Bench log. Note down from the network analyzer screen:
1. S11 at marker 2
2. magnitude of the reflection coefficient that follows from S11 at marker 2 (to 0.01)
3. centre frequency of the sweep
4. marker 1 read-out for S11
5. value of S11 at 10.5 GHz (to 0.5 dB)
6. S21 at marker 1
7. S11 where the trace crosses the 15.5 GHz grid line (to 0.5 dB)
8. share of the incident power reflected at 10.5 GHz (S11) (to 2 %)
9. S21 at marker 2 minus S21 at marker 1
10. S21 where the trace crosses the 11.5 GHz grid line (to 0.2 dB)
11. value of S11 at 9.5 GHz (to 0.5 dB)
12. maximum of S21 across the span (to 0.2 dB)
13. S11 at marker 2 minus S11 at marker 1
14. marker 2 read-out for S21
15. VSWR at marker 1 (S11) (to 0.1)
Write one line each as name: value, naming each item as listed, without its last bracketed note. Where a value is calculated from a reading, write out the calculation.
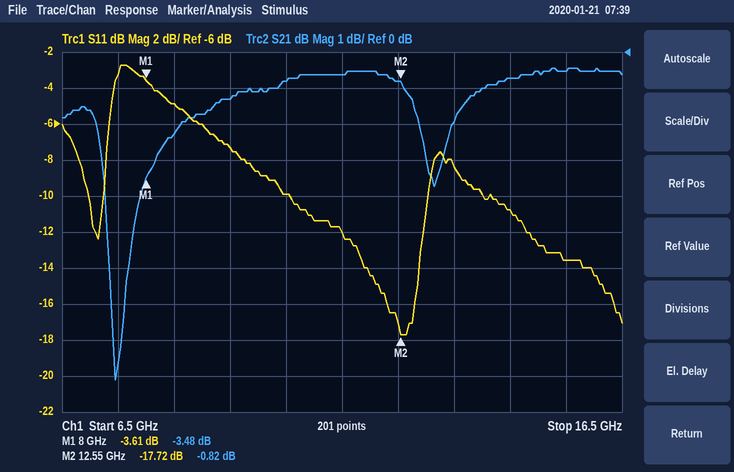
S11 at marker 2: -17.72 dB
magnitude of the reflection coefficient that follows from S11 at marker 2: 10^(-17.72/20) ≈ 0.13
centre frequency of the sweep: 11.5 GHz
marker 1 read-out for S11: -3.61 dB
value of S11 at 10.5 GHz: -10.0 dB
S21 at marker 1: -3.48 dB
S11 where the trace crosses the 15.5 GHz grid line: -13.5 dB
share of the incident power reflected at 10.5 GHz (S11): 10^(-10/10) ≈ 10 %
S21 at marker 2 minus S21 at marker 1: -0.82 − (-3.48) = 2.66 dB
S21 where the trace crosses the 11.5 GHz grid line: -0.6 dB
value of S11 at 9.5 GHz: -7.5 dB
maximum of S21 across the span: -0.4 dB
S11 at marker 2 minus S11 at marker 1: -17.72 − (-3.61) = -14.11 dB
marker 2 read-out for S21: -0.82 dB
VSWR at marker 1 (S11): (1 + 0.6599)/(1 − 0.6599) ≈ 4.9
